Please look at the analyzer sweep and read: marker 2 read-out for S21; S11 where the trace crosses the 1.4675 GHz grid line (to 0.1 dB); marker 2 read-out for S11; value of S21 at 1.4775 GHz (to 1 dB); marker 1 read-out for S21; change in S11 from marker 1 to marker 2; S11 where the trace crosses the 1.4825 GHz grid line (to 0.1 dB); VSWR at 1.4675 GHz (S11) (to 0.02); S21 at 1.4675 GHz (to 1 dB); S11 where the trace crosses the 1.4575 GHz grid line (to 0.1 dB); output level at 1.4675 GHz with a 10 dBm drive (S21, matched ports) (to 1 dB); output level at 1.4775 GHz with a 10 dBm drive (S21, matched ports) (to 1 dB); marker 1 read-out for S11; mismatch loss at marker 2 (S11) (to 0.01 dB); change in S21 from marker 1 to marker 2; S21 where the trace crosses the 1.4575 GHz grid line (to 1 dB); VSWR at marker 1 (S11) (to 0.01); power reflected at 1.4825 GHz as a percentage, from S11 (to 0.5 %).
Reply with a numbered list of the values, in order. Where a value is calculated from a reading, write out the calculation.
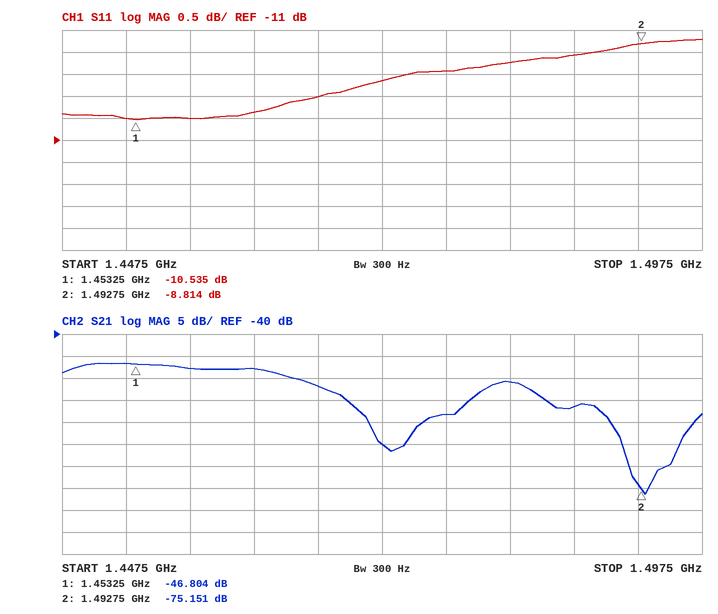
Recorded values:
1. -75.151 dB
2. -10.0 dB
3. -8.814 dB
4. -58 dB
5. -46.804 dB
6. -8.814 − (-10.535) = 1.721 dB
7. -9.2 dB
8. |Γ| = 10^(-10/20) = 0.3162; VSWR = (1 + 0.3162)/(1 − 0.3162) ≈ 1.92
9. -52 dB
10. -10.5 dB
11. 10 dBm + (-52 dB) = -42 dBm
12. 10 dBm + (-58 dB) = -48 dBm
13. -10.535 dB
14. −10 log10(1 − 10^(-8.814/10)) ≈ 0.61 dB
15. -75.151 − (-46.804) = -28.347 dB
16. -48 dB
17. (1 + 0.2973)/(1 − 0.2973) ≈ 1.85
18. 10^(-9.2/10) ≈ 12.0 %
